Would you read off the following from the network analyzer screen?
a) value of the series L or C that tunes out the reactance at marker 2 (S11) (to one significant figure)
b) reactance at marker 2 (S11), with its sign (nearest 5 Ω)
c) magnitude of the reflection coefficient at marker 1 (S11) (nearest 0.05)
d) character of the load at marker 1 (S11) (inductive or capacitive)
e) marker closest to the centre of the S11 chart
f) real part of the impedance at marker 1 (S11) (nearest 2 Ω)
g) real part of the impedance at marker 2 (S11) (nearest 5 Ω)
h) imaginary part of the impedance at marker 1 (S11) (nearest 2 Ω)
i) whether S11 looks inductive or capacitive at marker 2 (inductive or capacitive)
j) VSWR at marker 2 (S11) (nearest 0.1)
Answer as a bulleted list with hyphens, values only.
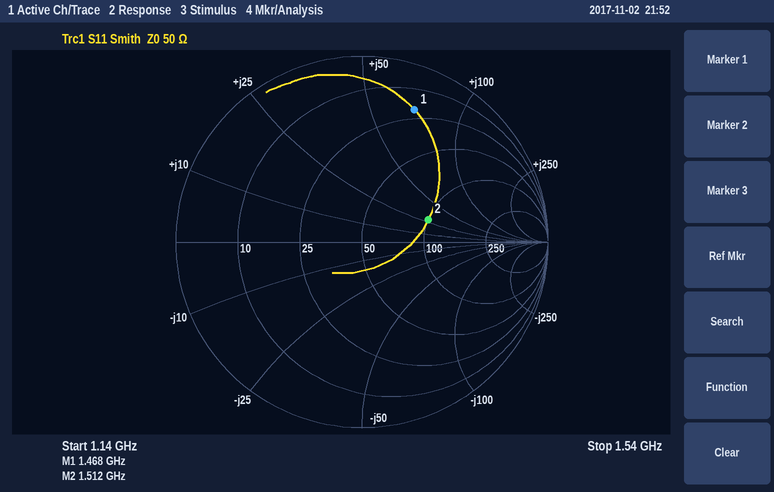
- 4 pF
- +30 Ω
- 0.75
- inductive
- marker 2
- 20 Ω
- 100 Ω
- +70 Ω
- inductive
- 2.2
